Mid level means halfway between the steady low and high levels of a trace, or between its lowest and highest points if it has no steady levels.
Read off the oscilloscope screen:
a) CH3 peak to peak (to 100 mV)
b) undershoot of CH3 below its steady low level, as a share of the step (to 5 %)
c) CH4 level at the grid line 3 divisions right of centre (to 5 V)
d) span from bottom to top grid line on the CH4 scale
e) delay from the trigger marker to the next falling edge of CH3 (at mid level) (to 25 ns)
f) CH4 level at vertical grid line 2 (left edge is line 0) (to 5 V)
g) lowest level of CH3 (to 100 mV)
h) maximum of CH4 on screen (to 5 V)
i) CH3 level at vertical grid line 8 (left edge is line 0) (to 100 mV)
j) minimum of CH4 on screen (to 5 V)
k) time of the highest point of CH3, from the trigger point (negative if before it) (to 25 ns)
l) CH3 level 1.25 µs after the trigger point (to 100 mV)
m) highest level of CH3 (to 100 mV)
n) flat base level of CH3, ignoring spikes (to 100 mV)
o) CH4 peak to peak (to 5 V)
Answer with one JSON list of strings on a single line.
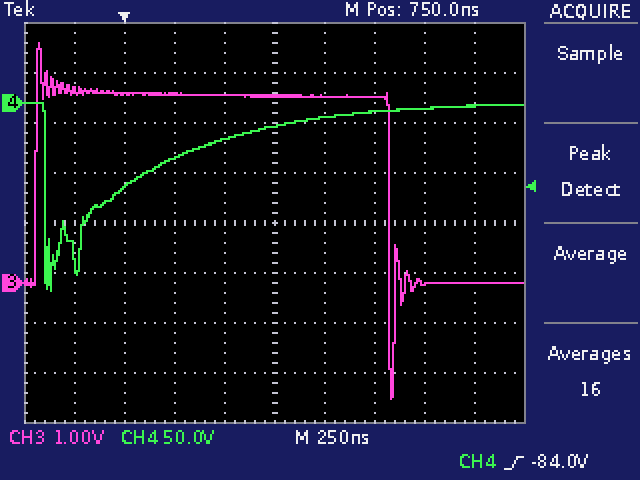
["7.1 V", "60 %", "-5 V", "400 V", "1.325 µs", "-85 V", "-2.3 V", "0 V", "0.0 V", "-190 V", "-425 ns", "3.7 V", "4.8 V", "0.0 V", "190 V"]
